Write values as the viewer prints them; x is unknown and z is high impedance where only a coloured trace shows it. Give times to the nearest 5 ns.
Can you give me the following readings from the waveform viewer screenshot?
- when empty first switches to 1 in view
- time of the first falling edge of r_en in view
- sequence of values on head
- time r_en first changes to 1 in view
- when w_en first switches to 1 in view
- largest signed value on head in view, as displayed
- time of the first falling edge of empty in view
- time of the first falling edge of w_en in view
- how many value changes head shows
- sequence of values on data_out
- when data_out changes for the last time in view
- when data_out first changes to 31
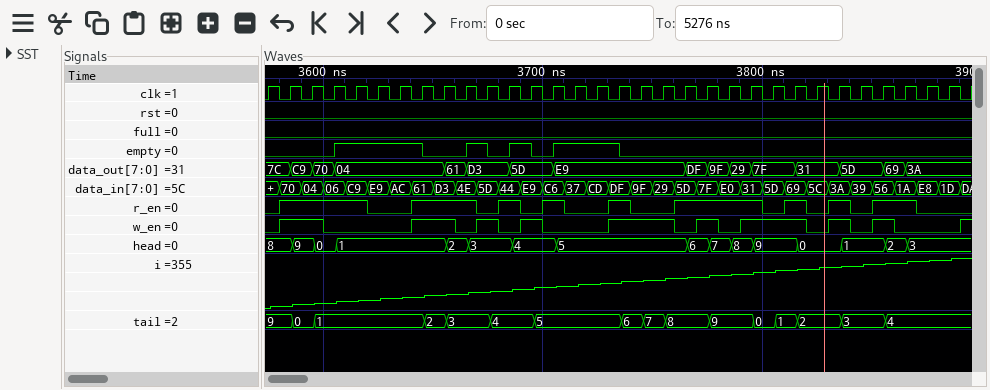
3605 ns
3620 ns
8, 9, 0, 1, 2, 3, 4, 5, 6, 7, 8, 9, 0, 1, 2, 3
3580 ns
3580 ns
9
3645 ns
3600 ns
15
7C, C9, 70, 04, 61, D3, 5D, E9, DF, 9F, 29, 7F, 31, 5D, 69, 3A
3865 ns
3815 ns
